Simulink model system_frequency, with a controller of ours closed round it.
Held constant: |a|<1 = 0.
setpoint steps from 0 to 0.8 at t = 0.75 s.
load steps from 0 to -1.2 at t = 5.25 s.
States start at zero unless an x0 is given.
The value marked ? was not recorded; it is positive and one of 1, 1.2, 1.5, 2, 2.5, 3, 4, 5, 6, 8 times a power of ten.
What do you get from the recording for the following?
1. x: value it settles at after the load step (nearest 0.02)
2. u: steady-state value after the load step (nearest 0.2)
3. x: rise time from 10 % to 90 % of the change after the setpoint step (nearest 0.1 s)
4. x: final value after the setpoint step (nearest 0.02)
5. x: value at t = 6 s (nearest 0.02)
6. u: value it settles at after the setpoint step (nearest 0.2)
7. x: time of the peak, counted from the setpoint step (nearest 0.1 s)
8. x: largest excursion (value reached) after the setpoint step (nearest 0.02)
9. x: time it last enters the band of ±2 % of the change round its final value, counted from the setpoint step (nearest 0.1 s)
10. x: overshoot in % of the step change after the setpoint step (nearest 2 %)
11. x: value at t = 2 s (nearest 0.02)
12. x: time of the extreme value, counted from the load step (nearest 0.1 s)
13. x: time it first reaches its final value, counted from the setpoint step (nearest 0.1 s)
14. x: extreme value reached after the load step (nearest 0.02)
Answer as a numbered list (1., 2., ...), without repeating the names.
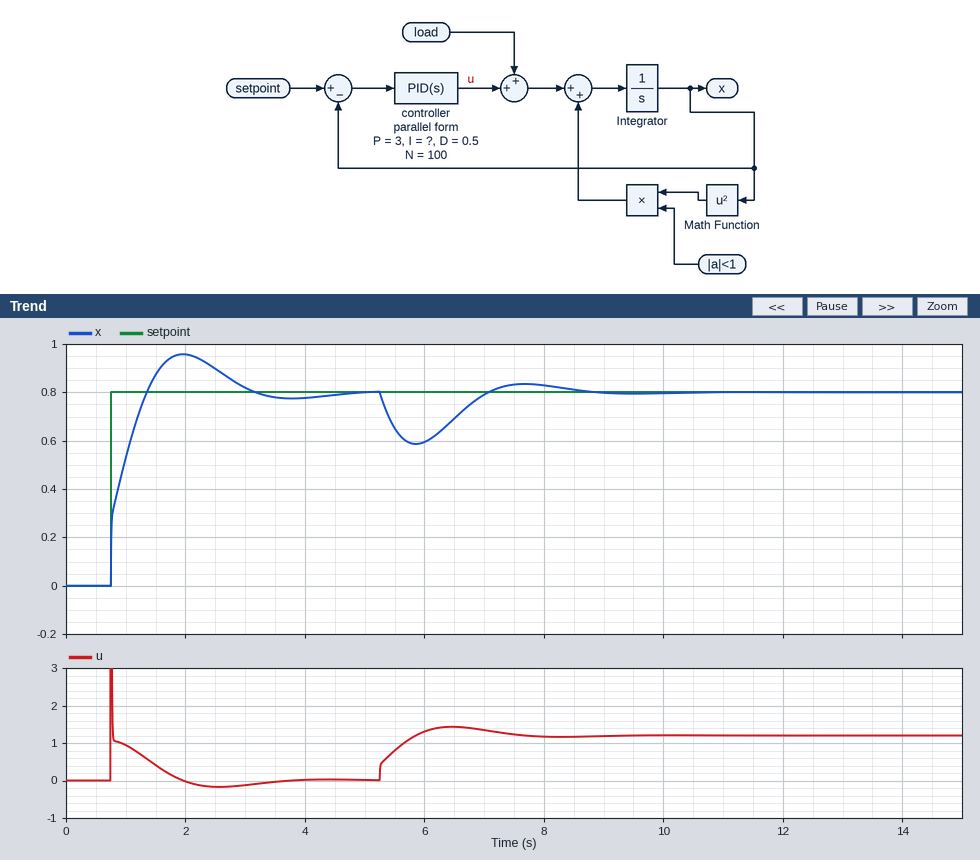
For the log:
1. 0.80
2. 1.2
3. 0.5 s
4. 0.80
5. 0.60
6. 0.0
7. 1.2 s
8. 0.96
9. 3.6 s
10. 20 %
11. 0.96
12. 0.6 s
13. 0.6 s
14. 0.58
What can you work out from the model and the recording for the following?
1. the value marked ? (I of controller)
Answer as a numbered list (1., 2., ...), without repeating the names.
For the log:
1. 6
